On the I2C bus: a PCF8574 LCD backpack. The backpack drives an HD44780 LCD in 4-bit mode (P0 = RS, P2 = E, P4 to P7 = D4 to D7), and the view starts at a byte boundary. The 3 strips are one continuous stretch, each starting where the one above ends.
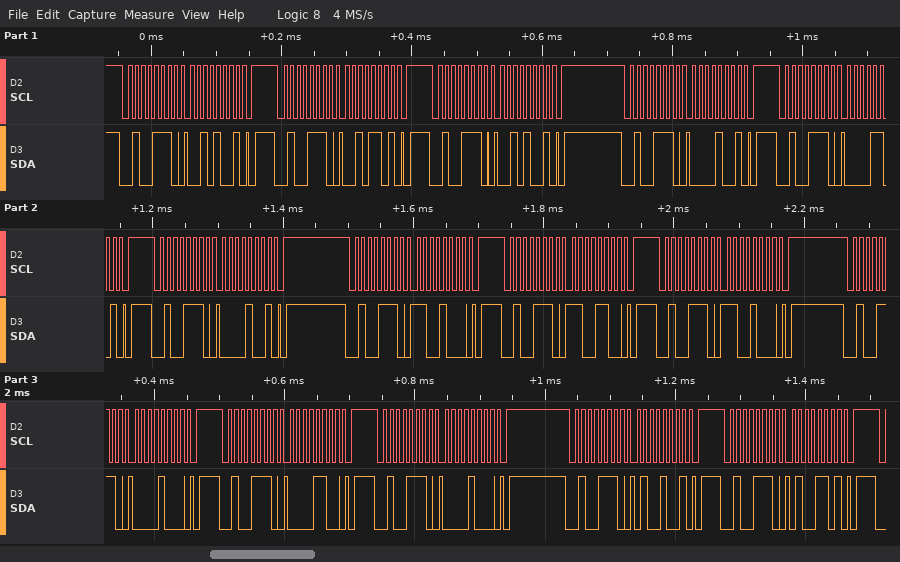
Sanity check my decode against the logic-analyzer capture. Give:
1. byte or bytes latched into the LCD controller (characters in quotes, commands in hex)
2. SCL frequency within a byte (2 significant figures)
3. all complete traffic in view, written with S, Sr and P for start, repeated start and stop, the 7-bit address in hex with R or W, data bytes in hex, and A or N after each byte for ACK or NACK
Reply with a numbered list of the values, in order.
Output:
1. ' ' 0xC0
2. 100 kHz
3. S 27W A 29 A P S 27W A 2D A P S 27W A 29 A P S 27W A 09 A P S 27W A 0D A P S 27W A 09 A P S 27W A C8 A P S 27W A CC A P S 27W A C8 A P S 27W A 08 A P S 27W A 0C A P S 27W A 08 A P S 27W A 49 A P S 27W A 4D A P
